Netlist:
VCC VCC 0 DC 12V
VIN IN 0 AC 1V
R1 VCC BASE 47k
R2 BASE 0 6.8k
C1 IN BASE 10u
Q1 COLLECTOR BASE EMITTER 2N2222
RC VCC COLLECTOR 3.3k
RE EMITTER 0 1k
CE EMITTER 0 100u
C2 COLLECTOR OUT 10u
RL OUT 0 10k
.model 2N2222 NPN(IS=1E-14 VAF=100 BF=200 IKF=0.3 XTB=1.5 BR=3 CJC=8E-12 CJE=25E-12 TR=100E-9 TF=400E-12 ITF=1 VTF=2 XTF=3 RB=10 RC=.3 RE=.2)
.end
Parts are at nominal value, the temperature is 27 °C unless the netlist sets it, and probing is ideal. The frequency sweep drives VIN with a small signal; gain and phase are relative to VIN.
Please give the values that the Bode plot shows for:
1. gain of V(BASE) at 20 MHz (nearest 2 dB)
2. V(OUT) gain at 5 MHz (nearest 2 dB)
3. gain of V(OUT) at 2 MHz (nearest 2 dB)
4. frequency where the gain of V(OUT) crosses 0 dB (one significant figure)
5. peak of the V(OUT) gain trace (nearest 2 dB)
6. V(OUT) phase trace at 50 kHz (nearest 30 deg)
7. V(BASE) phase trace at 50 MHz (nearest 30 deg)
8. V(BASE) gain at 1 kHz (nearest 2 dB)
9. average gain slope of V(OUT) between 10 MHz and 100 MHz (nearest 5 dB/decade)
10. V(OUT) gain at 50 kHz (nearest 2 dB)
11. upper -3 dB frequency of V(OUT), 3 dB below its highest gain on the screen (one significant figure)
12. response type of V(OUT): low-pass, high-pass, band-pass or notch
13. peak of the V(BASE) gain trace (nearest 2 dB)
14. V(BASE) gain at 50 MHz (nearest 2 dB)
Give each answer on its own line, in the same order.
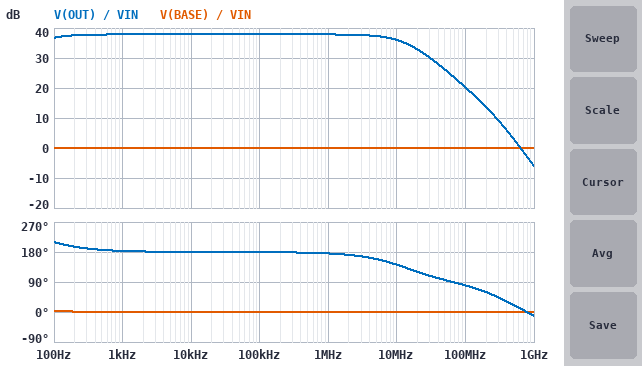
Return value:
0 dB
38 dB
38 dB
600 MHz
38 dB
180 deg
0 deg
0 dB
-15 dB/decade
38 dB
10 MHz
low-pass
0 dB
0 dB
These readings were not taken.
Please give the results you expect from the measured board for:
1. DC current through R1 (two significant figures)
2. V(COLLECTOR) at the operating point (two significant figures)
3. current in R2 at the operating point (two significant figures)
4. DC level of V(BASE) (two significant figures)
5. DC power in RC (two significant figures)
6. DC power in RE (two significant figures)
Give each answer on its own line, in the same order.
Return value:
220 µA
9.2 V
220 µA
1.5 V
2.3 mW
710 µW
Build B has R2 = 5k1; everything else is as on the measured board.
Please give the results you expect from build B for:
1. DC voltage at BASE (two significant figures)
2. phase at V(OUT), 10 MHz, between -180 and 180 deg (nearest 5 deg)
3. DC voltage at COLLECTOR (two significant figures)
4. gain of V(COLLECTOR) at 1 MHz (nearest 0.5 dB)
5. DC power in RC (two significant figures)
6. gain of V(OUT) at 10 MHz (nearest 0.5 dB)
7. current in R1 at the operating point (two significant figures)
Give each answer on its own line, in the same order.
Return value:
1.2 V
145 deg
10 V
34.0 dB
910 µW
32.5 dB
230 µA
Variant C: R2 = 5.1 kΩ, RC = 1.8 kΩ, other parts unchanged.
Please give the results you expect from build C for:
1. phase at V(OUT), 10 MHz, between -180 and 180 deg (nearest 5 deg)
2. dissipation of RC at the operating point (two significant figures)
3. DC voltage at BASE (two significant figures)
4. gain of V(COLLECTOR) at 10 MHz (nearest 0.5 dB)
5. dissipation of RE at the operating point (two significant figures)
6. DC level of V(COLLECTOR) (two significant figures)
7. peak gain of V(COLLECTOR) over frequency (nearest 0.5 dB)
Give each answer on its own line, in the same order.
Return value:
155 deg
500 µW
1.2 V
29.0 dB
280 µW
11 V
29.5 dB
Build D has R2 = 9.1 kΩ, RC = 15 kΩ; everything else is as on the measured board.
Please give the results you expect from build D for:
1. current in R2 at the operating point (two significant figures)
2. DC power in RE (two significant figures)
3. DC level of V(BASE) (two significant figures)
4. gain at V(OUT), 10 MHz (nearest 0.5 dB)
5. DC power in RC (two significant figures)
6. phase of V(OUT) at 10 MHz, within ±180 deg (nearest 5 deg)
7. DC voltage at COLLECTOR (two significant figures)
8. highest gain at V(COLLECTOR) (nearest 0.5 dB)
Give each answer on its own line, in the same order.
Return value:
160 µA
650 µW
1.5 V
-1.5 dB
8.3 mW
40 deg
850 mV
9.0 dB
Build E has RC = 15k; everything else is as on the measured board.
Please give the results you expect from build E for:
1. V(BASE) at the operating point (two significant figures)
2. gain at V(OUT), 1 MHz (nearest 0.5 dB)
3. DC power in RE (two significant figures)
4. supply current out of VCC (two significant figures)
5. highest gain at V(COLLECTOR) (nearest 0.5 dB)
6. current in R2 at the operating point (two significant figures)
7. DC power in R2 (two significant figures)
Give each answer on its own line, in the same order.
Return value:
1.4 V
20.0 dB
580 µW
970 µA
21.5 dB
210 µA
290 µW
